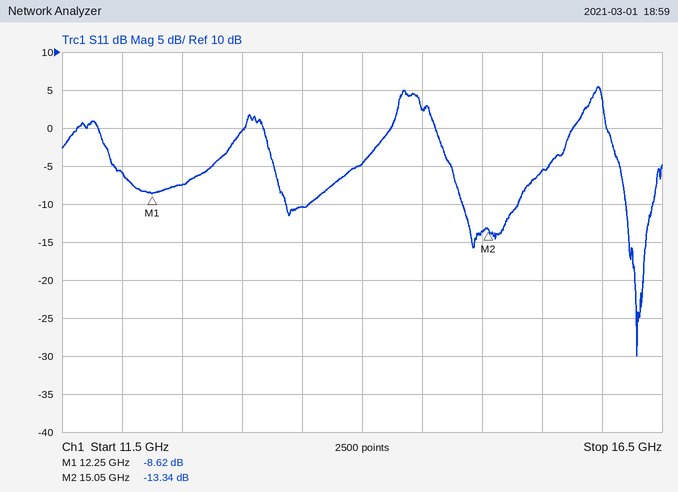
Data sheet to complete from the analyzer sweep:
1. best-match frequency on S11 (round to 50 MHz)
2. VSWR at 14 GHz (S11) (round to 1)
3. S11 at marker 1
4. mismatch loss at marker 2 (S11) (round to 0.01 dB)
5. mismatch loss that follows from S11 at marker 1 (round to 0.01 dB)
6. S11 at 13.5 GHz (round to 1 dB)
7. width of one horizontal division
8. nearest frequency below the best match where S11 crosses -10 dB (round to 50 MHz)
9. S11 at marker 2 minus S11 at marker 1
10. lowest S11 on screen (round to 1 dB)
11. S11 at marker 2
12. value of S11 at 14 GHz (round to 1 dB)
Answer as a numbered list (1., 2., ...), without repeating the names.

1. 16.30 GHz
2. 4
3. -8.62 dB
4. 0.21 dB
5. 0.64 dB
6. -10 dB
7. 500 MHz
8. 16.20 GHz
9. -4.72 dB
10. -30 dB
11. -13.34 dB
12. -5 dB
